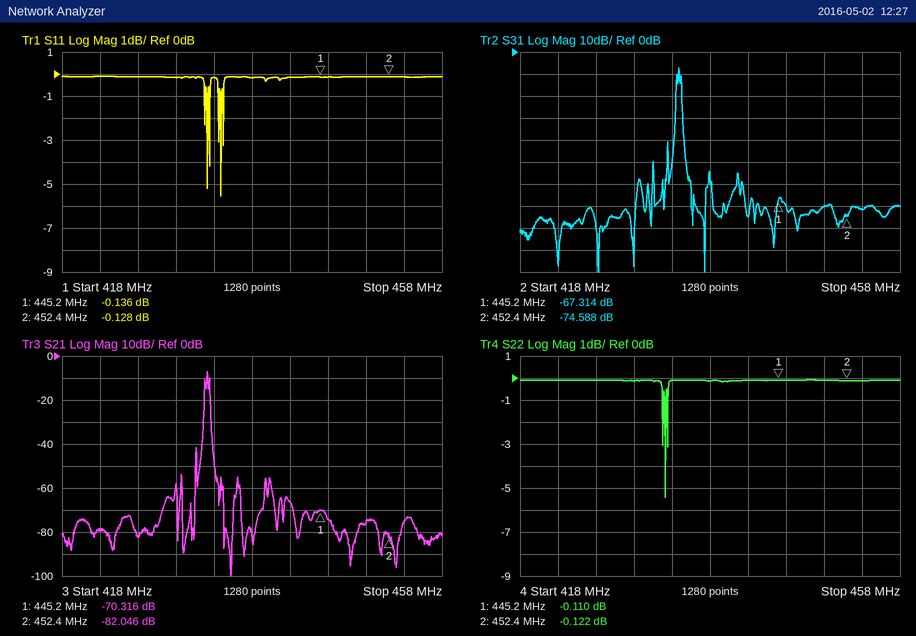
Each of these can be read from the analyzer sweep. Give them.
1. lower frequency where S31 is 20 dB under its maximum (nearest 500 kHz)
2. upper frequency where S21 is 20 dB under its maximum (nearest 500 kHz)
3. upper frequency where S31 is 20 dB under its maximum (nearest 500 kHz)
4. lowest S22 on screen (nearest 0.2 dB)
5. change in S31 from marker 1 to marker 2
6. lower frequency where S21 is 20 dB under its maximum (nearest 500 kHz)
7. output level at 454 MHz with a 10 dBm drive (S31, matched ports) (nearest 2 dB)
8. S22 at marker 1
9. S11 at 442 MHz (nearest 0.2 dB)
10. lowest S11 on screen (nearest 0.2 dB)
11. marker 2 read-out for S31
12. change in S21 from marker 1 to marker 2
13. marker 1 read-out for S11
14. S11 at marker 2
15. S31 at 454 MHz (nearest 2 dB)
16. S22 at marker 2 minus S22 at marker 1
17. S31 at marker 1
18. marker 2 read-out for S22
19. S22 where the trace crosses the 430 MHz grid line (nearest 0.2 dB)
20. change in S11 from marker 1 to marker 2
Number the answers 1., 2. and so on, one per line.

1. 434.5 MHz
2. 433.5 MHz
3. 435.0 MHz
4. -5.4 dB
5. -7.274 dB
6. 433.0 MHz
7. -62 dBm
8. -0.110 dB
9. -0.2 dB
10. -5.6 dB
11. -74.588 dB
12. -11.730 dB
13. -0.136 dB
14. -0.128 dB
15. -72 dB
16. -0.012 dB
17. -67.314 dB
18. -0.122 dB
19. -0.2 dB
20. 0.008 dB
